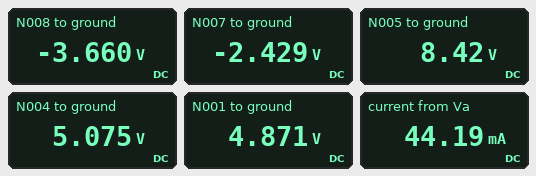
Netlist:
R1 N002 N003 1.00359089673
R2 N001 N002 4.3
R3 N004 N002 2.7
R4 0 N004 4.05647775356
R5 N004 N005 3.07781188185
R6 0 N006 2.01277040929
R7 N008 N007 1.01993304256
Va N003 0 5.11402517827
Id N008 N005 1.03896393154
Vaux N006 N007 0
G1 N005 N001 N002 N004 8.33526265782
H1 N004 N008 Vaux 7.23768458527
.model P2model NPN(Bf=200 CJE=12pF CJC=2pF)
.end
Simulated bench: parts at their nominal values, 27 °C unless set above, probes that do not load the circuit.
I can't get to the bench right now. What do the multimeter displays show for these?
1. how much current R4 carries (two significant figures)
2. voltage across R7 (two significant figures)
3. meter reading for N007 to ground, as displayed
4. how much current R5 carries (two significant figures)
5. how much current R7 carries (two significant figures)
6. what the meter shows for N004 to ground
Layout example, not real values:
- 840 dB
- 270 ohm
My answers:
- 1.3 A
- 1.2 V
- -2.429 V
- 1.1 A
- 1.2 A
- 5.075 V
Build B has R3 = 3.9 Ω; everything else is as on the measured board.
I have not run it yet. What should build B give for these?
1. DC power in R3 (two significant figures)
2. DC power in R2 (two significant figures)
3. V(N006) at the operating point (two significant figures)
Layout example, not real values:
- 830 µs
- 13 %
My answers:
- 7.7 µW
- 8.9 mW
- -2.4 V
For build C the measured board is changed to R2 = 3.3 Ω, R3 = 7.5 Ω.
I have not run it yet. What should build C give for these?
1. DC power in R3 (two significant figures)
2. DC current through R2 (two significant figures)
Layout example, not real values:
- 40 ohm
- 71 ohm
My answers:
- 3.9 µW
- 45 mA
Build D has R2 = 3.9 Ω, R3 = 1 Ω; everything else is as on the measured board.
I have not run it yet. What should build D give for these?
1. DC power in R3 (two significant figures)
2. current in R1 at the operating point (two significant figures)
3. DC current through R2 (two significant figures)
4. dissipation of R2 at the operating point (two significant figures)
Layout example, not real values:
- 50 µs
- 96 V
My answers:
- 36 µW
- 44 mA
- 50 mA
- 9.8 mW
